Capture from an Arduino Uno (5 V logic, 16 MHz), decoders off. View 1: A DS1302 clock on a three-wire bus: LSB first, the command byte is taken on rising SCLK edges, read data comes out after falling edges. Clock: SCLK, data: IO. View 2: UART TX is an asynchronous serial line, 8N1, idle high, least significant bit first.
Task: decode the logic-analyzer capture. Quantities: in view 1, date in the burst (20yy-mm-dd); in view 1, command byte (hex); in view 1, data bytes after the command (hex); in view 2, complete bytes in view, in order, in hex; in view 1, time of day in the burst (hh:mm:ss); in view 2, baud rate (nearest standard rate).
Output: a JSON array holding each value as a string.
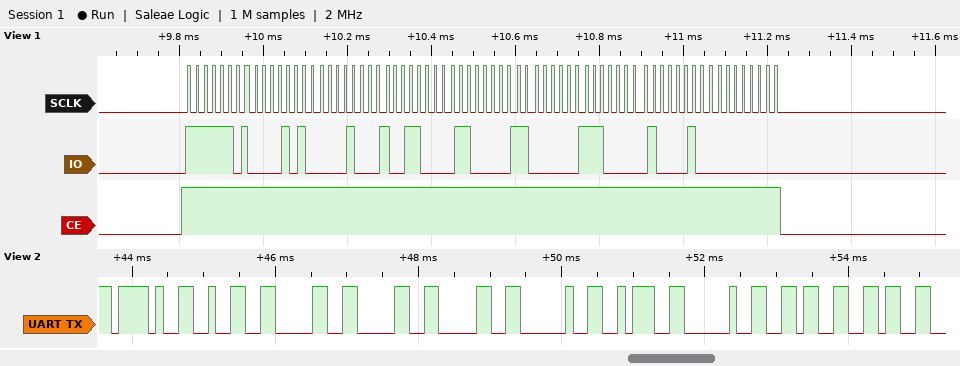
["2021-03-06", "0xBF", "50 10 19 06 03 07 21 00", "0x2F 0x32 0x30 0x30 0x30 0x20 0x3A 0x20 0x36 0x36", "19:10:50", "9600 baud"]
